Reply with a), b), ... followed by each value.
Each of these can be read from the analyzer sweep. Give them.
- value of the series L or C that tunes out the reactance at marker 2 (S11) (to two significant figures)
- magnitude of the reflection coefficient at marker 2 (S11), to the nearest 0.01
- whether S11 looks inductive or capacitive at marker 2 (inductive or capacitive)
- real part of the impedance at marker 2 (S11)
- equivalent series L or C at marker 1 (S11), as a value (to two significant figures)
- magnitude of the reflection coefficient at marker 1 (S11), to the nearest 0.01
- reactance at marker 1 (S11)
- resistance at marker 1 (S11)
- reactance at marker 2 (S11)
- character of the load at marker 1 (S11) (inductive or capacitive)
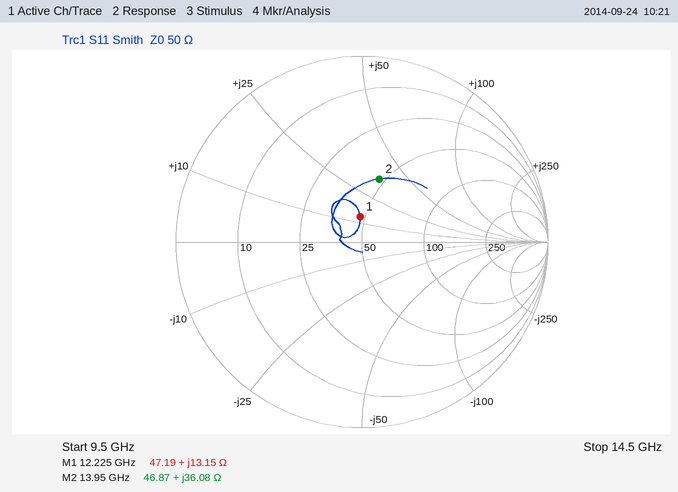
a) 320 fF
b) 0.35
c) inductive
d) 46.87 Ω
e) 170 pH
f) 0.14
g) +13.15 Ω
h) 47.19 Ω
i) +36.08 Ω
j) inductive
